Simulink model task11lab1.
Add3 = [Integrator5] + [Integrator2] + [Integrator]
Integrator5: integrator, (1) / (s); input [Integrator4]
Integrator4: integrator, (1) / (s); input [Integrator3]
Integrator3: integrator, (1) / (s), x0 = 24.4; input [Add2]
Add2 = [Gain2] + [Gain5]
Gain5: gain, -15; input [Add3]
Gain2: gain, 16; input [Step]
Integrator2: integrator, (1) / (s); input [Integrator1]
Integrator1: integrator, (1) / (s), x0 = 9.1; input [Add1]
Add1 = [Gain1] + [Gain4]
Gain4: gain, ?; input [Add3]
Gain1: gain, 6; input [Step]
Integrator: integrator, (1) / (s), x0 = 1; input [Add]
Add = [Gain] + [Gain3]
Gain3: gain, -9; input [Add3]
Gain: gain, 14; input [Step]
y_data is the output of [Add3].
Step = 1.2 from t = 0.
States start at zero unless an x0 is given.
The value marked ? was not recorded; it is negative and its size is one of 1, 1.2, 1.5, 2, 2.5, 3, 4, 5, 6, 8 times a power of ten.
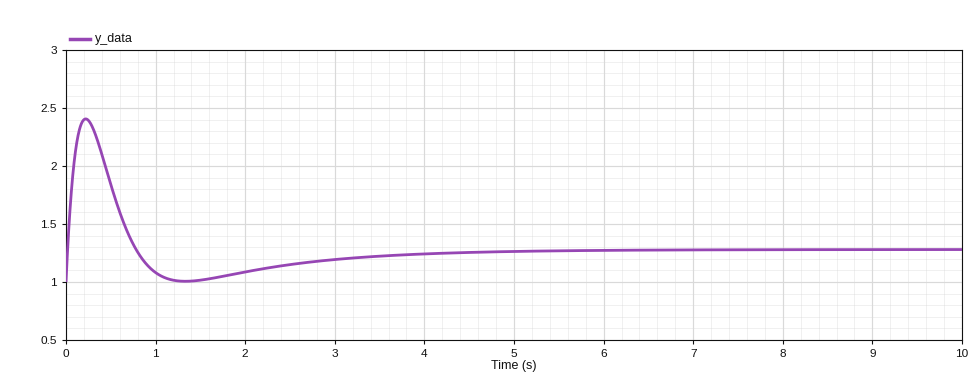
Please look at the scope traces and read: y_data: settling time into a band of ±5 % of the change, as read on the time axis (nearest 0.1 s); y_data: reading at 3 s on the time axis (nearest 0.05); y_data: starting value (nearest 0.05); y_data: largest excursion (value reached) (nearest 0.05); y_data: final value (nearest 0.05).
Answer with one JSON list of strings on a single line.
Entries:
["5.2 s", "1.20", "1.00", "2.40", "1.30"]
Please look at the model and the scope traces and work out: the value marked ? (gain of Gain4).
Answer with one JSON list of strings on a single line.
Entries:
["-25"]
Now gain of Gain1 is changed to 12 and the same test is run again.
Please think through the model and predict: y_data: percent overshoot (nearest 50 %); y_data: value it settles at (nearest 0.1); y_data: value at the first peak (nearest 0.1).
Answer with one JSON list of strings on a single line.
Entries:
["450 %", "1.3", "2.5"]
